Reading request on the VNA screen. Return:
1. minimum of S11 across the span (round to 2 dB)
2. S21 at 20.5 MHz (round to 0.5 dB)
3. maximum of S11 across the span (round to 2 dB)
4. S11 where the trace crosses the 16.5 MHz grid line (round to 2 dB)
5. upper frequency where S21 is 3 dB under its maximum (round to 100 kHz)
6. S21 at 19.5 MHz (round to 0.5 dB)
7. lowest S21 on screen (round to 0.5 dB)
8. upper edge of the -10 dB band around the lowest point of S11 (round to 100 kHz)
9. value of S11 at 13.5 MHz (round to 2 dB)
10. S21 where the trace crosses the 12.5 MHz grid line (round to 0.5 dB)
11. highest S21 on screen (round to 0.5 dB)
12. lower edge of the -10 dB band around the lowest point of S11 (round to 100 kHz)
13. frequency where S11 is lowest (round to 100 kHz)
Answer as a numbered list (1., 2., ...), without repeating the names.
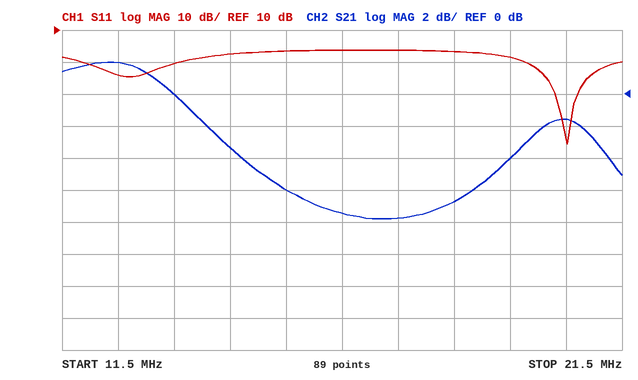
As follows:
1. -26 dB
2. -1.5 dB
3. 4 dB
4. 4 dB
5. 13.8 MHz
6. -4.0 dB
7. -8.0 dB
8. 20.7 MHz
9. 0 dB
10. 2.0 dB
11. 2.0 dB
12. 20.3 MHz
13. 20.5 MHz
